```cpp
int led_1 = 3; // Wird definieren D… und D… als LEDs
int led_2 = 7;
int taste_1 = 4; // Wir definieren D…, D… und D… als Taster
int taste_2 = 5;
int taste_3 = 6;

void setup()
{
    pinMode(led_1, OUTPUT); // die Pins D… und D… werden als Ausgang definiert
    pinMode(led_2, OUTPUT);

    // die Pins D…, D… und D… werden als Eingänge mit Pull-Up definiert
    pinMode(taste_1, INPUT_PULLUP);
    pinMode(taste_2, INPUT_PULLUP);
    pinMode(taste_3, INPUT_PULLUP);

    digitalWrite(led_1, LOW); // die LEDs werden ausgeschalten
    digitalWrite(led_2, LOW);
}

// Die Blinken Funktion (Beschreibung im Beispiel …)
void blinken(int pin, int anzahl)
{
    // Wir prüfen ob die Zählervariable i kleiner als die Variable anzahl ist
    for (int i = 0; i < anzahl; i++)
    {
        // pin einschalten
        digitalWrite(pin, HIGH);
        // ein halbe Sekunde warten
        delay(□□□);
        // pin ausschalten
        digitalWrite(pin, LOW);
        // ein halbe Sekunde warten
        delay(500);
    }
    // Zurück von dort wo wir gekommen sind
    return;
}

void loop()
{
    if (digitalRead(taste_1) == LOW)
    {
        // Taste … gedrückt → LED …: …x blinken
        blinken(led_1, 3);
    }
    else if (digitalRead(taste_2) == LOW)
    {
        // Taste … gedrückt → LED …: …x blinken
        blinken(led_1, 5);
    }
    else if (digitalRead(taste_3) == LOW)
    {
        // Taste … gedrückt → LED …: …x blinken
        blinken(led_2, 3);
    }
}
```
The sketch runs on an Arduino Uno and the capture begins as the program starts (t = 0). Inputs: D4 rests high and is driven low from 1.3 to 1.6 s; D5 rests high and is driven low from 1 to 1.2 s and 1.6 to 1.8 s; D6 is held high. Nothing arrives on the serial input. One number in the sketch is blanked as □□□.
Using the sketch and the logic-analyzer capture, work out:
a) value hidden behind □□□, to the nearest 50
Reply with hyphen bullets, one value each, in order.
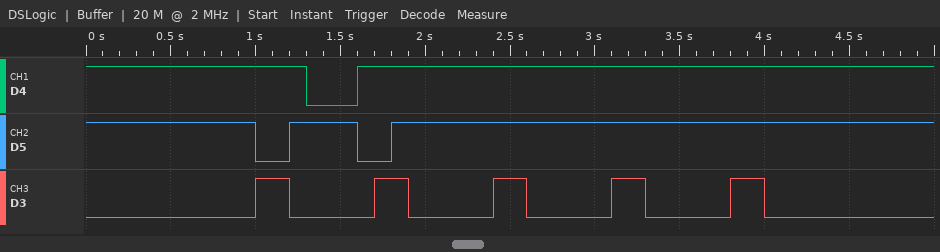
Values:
- 200
